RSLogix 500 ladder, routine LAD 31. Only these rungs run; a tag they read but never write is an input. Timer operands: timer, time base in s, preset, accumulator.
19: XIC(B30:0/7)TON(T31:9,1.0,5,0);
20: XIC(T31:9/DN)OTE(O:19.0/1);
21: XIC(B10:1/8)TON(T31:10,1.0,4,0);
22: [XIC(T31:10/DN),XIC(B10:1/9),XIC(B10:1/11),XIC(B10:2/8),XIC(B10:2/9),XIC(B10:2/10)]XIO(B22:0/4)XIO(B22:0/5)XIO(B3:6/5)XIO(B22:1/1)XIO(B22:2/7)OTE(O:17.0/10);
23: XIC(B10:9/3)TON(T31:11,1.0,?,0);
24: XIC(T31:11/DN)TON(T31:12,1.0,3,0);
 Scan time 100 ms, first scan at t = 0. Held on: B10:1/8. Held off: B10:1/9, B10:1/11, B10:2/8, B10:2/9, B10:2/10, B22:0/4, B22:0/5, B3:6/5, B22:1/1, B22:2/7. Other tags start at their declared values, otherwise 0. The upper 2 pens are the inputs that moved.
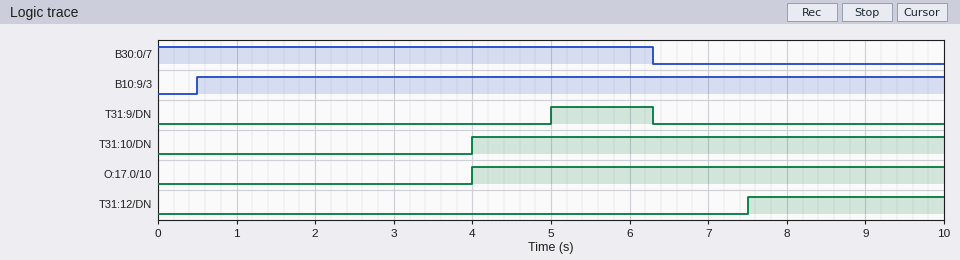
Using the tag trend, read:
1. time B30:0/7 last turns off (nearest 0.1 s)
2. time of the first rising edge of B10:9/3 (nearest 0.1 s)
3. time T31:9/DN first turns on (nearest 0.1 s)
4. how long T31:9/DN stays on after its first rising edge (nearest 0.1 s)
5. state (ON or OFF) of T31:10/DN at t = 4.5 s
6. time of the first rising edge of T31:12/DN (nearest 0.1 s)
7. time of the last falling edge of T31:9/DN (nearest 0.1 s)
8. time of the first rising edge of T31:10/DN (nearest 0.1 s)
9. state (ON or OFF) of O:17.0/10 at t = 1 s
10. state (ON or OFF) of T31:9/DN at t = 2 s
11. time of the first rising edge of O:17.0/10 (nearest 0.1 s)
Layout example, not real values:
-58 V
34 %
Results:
6.3 s
0.5 s
5.0 s
1.3 s
ON
7.5 s
6.3 s
4.0 s
OFF
OFF
4.0 s
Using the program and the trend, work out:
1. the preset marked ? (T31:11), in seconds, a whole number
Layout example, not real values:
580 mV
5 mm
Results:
4 s
